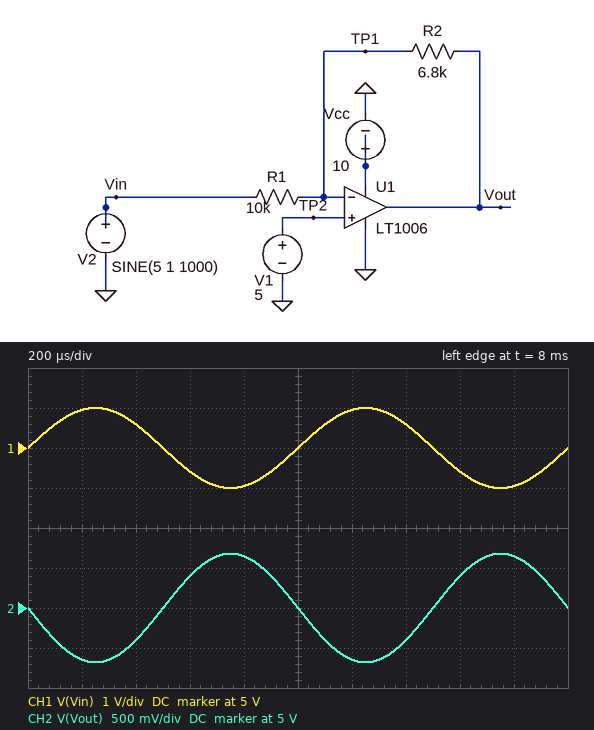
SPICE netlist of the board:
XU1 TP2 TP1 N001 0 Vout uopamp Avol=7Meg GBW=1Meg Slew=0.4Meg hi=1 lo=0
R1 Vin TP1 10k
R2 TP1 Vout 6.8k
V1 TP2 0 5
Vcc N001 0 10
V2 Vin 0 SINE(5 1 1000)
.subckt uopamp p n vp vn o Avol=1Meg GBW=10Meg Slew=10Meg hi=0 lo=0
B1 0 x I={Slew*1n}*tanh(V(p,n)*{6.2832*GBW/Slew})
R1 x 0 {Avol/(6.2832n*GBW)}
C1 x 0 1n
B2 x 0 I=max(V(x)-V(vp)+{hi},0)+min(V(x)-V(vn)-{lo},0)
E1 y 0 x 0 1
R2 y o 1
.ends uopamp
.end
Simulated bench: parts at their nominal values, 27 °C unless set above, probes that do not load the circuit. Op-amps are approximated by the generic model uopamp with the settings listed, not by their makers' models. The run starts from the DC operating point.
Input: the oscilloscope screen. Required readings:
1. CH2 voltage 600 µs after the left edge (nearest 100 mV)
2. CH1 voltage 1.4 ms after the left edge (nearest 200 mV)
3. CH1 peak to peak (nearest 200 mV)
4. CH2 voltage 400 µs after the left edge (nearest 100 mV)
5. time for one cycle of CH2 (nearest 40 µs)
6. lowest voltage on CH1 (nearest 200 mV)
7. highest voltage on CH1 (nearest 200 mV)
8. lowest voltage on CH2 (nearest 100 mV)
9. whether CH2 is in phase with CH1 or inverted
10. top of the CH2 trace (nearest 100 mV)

5.4 V
5.6 V
2.0 V
4.6 V
1.00 ms
4.0 V
6.0 V
4.3 V
inverted
5.7 V
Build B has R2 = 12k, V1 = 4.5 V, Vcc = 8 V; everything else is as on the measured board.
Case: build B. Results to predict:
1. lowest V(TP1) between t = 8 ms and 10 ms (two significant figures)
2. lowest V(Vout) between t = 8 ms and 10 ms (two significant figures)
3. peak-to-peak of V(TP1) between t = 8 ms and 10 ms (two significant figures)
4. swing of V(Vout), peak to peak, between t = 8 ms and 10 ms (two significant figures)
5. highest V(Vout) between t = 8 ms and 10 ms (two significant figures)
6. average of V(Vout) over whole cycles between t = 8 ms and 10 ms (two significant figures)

4.5 V
2.7 V
2.4 mV
2.4 V
5.1 V
3.9 V
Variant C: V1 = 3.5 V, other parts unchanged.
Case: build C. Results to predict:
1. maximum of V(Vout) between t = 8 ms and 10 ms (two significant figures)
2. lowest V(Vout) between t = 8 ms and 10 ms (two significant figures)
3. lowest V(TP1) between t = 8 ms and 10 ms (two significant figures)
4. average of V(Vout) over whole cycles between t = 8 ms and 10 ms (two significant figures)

3.2 V
1.8 V
3.5 V
2.5 V
